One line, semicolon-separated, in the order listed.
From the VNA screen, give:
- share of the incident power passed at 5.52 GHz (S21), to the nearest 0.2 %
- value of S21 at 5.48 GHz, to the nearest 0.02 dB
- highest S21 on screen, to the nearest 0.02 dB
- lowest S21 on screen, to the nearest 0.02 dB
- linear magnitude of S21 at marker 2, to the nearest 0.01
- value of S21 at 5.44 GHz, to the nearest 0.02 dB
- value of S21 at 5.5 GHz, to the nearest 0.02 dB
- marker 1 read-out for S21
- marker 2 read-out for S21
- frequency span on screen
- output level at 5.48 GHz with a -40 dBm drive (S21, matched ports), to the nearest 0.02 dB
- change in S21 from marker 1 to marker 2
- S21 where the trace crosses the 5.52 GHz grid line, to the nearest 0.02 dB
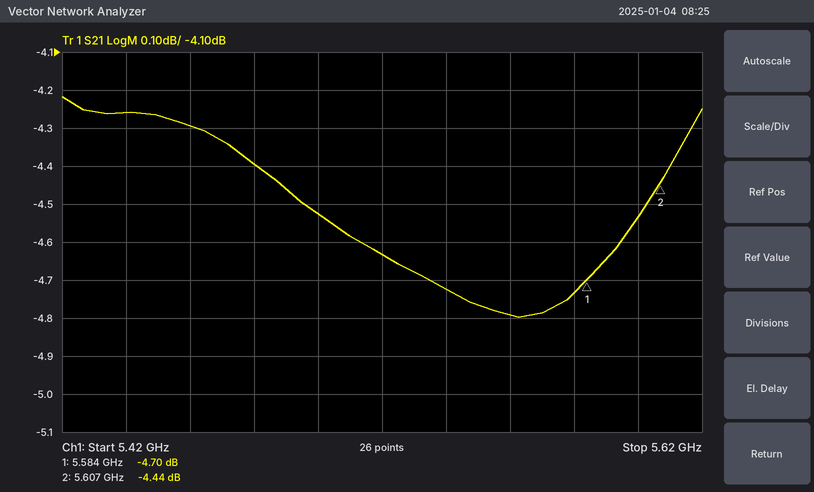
34.4 %; -4.40 dB; -4.22 dB; -4.80 dB; 0.60; -4.26 dB; -4.52 dB; -4.70 dB; -4.44 dB; 200 MHz; -44.40 dBm; 0.26 dB; -4.64 dB
